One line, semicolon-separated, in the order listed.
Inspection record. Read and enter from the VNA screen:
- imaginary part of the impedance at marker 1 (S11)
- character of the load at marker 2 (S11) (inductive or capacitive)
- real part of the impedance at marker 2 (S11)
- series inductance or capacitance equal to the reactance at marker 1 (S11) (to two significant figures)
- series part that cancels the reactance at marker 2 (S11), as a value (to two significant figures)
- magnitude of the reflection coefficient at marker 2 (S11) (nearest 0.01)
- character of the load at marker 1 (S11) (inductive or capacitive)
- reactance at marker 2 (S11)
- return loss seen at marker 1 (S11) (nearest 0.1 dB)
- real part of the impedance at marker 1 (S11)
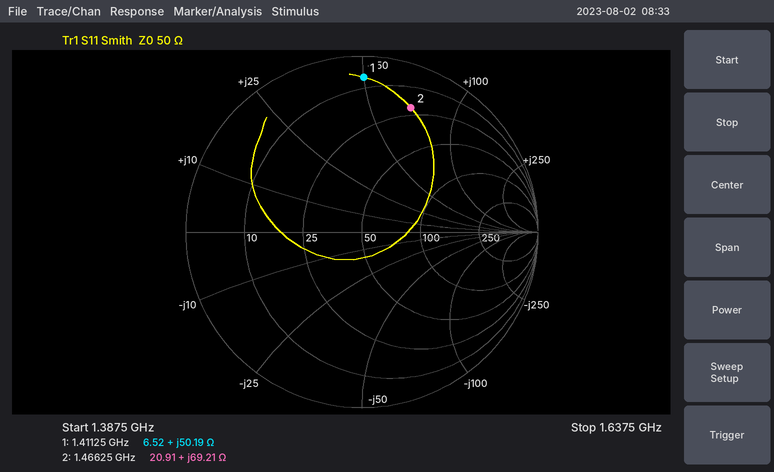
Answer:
+50.19 Ω; inductive; 20.91 Ω; 5.7 nH; 1.6 pF; 0.76; inductive; +69.21 Ω; 1.1 dB; 6.52 Ω
